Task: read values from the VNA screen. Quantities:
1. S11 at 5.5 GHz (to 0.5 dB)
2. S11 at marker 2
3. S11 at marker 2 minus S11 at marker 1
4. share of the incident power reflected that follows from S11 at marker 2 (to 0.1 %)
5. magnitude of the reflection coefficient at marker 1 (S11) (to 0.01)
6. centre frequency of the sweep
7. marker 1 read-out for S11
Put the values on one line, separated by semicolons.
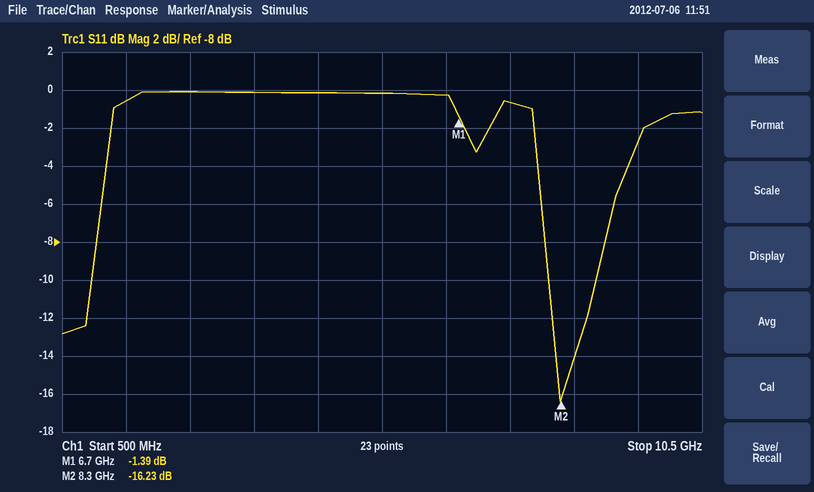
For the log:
0.0 dB; -16.23 dB; -14.84 dB; 2.4 %; 0.85; 5.5 GHz; -1.39 dB
